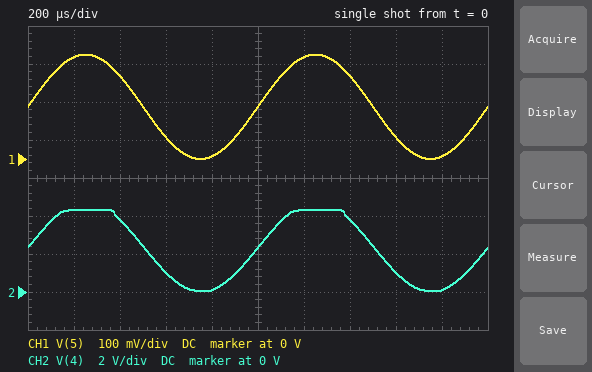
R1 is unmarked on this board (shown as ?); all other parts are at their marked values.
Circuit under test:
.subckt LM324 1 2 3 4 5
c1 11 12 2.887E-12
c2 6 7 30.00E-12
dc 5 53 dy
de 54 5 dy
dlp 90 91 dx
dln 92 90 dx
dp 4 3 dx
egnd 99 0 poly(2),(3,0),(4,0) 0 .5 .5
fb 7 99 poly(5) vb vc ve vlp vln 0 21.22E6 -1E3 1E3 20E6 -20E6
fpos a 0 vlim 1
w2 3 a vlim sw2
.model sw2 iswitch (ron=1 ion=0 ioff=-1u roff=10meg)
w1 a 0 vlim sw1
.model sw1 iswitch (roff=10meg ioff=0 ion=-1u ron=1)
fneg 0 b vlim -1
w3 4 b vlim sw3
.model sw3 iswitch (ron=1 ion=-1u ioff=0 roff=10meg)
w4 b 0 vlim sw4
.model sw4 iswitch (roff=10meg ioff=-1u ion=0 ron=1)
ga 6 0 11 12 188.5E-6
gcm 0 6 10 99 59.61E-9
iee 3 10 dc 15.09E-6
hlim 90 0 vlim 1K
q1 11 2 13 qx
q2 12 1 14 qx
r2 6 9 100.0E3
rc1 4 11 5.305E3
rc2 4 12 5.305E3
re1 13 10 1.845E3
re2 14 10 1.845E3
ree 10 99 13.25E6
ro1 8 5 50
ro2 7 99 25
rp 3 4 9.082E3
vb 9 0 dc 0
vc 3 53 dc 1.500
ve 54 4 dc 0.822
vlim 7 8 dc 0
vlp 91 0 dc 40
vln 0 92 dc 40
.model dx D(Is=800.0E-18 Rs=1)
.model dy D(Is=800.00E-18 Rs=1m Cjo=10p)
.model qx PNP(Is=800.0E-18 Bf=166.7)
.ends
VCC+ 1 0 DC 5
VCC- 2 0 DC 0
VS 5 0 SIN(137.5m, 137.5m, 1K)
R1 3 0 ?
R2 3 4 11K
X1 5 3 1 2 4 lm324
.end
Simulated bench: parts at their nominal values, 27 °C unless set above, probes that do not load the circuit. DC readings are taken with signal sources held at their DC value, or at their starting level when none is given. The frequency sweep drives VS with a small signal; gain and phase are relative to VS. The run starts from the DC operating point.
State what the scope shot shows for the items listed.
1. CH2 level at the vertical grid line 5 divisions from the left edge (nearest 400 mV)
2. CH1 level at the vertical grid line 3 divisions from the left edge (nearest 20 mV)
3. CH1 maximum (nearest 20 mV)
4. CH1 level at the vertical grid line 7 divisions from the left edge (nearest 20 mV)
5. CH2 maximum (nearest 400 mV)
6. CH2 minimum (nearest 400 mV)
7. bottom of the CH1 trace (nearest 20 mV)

2.4 V
60 mV
280 mV
220 mV
4.4 V
0 V
0 V
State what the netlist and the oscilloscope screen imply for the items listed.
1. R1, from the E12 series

680 Ω
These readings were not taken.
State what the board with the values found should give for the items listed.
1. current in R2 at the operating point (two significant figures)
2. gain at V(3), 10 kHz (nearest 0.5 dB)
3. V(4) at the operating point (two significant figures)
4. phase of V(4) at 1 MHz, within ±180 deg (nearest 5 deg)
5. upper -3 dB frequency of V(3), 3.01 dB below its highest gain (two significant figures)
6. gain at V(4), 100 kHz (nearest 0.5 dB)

200 µA
0 dB
2.4 V
-100 deg
59 kHz
19.0 dB
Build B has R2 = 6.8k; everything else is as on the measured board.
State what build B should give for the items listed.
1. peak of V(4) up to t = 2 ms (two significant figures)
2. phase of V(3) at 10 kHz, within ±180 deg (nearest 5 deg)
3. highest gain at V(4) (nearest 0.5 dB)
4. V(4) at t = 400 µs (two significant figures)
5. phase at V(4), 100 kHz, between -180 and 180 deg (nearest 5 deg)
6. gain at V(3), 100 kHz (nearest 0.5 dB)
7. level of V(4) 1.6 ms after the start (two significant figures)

3.0 V
-5 deg
21.0 dB
2.4 V
-50 deg
-3.5 dB
640 mV
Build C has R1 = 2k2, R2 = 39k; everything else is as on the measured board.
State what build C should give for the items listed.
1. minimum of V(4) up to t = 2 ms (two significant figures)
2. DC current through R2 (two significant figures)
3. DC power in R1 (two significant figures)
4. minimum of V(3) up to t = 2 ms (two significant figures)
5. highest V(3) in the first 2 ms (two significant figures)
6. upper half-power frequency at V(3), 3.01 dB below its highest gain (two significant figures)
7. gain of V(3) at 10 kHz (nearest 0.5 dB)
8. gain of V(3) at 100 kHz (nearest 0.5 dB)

52 mV
63 µA
8.7 µW
2.9 mV
230 mV
54 kHz
0 dB
-6.5 dB
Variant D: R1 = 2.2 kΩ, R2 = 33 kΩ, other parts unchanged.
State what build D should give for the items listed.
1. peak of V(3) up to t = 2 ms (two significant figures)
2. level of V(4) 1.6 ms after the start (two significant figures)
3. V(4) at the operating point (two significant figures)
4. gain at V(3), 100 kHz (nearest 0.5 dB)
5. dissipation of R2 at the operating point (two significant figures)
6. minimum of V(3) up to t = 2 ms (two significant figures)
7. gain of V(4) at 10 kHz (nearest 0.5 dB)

270 mV
940 mV
2.2 V
-5.5 dB
130 µW
3.1 mV
24.0 dB
